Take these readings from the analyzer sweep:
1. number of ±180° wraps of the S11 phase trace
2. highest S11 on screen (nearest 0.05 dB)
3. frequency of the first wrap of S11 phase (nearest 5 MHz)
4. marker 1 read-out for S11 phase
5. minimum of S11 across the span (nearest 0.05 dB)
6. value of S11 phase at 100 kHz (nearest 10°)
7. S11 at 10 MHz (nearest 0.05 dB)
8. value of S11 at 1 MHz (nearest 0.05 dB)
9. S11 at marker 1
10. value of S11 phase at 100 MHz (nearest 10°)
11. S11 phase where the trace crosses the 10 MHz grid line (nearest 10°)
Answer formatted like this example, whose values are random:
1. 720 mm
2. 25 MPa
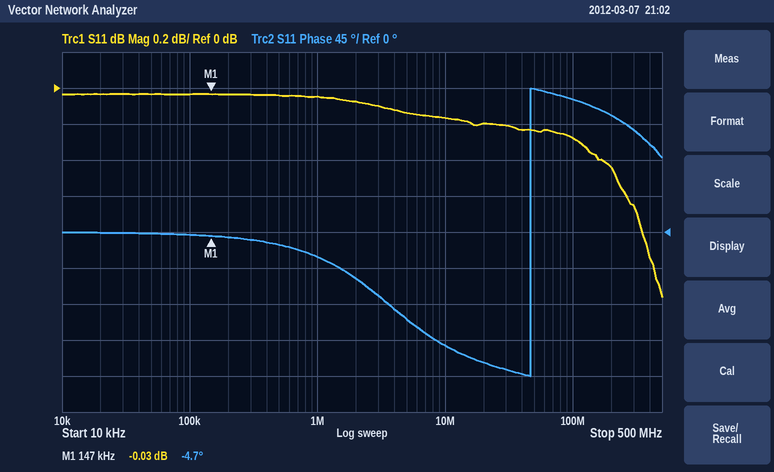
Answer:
1. 1
2. -0.05 dB
3. 45 MHz
4. -4.7°
5. -1.15 dB
6. 0°
7. -0.15 dB
8. -0.05 dB
9. -0.03 dB
10. 170°
11. -140°
